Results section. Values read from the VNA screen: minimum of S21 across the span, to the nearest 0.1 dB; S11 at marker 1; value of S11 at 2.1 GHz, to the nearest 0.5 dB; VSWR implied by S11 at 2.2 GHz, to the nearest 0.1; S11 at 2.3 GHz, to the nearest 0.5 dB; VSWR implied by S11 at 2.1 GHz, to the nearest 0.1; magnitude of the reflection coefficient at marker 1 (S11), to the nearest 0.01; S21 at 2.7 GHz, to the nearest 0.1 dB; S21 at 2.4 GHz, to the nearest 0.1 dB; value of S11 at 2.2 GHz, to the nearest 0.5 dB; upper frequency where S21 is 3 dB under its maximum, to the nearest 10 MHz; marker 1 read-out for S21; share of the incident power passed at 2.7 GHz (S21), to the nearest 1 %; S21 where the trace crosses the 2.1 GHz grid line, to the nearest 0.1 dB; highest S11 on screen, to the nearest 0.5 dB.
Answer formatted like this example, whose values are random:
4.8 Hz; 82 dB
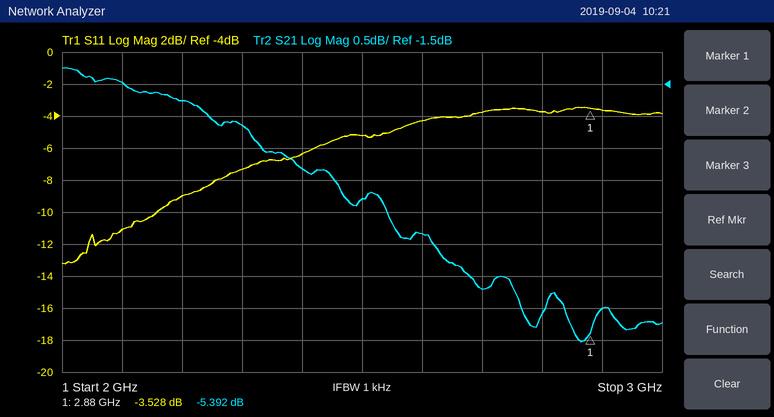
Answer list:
-5.5 dB; -3.528 dB; -11.0 dB; 2.1; -7.5 dB; 1.8; 0.67; -4.7 dB; -2.8 dB; -9.0 dB; 2.64 GHz; -5.392 dB; 34 %; -1.5 dB; -3.5 dB
